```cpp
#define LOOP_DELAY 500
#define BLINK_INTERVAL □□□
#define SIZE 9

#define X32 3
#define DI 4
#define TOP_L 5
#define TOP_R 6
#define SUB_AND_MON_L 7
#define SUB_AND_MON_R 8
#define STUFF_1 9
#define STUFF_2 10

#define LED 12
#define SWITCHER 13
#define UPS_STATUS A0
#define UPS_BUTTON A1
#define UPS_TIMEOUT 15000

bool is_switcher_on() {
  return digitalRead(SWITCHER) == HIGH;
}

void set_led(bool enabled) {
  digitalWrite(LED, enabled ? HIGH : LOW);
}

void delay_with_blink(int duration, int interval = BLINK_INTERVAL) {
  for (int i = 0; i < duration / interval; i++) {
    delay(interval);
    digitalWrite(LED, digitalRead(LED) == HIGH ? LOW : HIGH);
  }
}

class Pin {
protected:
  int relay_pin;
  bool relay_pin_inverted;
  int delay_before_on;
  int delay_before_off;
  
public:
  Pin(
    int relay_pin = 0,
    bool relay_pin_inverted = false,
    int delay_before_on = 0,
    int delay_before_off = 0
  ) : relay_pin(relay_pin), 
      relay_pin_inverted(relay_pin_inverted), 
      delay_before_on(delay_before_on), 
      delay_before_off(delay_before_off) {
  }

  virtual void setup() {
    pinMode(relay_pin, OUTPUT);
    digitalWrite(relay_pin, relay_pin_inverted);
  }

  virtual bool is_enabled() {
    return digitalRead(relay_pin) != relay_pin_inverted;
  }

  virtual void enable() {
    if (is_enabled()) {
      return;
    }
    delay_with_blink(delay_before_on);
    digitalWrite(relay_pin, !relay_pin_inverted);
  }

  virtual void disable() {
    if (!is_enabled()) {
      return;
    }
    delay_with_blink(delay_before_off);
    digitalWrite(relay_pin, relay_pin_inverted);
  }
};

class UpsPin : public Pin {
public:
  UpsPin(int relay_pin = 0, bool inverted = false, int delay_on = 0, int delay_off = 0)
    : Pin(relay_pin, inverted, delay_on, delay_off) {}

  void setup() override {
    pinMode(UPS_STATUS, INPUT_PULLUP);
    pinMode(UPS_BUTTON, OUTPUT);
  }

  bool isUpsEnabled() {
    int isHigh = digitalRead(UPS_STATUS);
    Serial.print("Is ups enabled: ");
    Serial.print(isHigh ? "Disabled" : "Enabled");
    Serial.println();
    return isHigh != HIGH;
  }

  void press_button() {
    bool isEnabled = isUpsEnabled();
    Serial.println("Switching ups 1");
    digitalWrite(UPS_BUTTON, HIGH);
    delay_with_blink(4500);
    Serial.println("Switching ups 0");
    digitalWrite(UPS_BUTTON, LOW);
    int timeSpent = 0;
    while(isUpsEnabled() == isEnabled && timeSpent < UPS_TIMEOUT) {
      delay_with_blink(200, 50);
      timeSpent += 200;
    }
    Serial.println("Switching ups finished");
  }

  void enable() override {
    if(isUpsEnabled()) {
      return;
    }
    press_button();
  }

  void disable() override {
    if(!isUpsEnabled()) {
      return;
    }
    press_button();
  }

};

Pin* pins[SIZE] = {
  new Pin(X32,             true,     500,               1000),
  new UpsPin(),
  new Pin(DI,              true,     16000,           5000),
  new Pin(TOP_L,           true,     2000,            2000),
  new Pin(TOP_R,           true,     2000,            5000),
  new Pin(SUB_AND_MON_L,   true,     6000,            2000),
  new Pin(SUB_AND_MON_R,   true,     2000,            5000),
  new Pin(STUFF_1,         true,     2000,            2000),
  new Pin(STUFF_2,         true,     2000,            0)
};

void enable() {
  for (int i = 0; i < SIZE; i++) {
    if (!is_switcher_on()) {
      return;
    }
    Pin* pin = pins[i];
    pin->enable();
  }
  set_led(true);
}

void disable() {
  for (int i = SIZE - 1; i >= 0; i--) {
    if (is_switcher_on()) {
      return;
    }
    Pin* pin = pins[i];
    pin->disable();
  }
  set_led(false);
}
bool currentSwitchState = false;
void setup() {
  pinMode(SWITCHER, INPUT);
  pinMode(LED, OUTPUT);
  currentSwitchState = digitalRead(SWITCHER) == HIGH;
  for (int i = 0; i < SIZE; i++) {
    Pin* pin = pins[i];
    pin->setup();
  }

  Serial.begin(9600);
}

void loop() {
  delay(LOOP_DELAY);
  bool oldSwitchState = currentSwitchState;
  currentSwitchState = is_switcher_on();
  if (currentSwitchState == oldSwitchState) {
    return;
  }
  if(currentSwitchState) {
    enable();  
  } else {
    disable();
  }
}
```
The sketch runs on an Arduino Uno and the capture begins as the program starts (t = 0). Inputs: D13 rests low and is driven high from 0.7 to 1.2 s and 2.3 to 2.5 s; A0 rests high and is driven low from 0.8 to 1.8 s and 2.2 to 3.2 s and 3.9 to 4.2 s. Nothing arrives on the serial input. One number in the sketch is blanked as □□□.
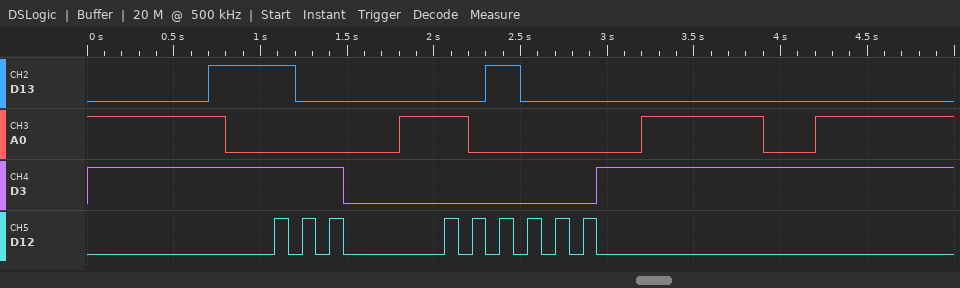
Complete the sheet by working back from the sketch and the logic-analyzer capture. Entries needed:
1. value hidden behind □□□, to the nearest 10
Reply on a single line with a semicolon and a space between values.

80
